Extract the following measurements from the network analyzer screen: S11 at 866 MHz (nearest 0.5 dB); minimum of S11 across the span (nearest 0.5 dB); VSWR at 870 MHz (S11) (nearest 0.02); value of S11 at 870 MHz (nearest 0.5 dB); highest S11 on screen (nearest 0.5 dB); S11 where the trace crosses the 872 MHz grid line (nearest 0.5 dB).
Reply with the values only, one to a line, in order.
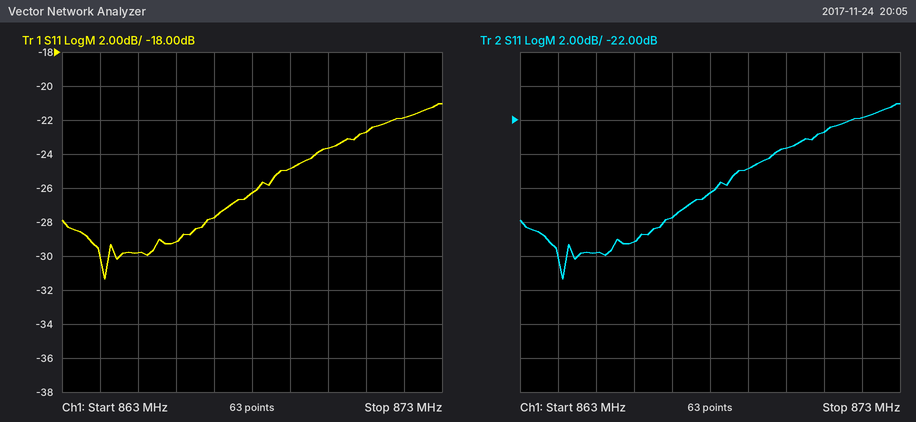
-29.0 dB
-31.5 dB
1.14
-23.5 dB
-21.0 dB
-22.0 dB
